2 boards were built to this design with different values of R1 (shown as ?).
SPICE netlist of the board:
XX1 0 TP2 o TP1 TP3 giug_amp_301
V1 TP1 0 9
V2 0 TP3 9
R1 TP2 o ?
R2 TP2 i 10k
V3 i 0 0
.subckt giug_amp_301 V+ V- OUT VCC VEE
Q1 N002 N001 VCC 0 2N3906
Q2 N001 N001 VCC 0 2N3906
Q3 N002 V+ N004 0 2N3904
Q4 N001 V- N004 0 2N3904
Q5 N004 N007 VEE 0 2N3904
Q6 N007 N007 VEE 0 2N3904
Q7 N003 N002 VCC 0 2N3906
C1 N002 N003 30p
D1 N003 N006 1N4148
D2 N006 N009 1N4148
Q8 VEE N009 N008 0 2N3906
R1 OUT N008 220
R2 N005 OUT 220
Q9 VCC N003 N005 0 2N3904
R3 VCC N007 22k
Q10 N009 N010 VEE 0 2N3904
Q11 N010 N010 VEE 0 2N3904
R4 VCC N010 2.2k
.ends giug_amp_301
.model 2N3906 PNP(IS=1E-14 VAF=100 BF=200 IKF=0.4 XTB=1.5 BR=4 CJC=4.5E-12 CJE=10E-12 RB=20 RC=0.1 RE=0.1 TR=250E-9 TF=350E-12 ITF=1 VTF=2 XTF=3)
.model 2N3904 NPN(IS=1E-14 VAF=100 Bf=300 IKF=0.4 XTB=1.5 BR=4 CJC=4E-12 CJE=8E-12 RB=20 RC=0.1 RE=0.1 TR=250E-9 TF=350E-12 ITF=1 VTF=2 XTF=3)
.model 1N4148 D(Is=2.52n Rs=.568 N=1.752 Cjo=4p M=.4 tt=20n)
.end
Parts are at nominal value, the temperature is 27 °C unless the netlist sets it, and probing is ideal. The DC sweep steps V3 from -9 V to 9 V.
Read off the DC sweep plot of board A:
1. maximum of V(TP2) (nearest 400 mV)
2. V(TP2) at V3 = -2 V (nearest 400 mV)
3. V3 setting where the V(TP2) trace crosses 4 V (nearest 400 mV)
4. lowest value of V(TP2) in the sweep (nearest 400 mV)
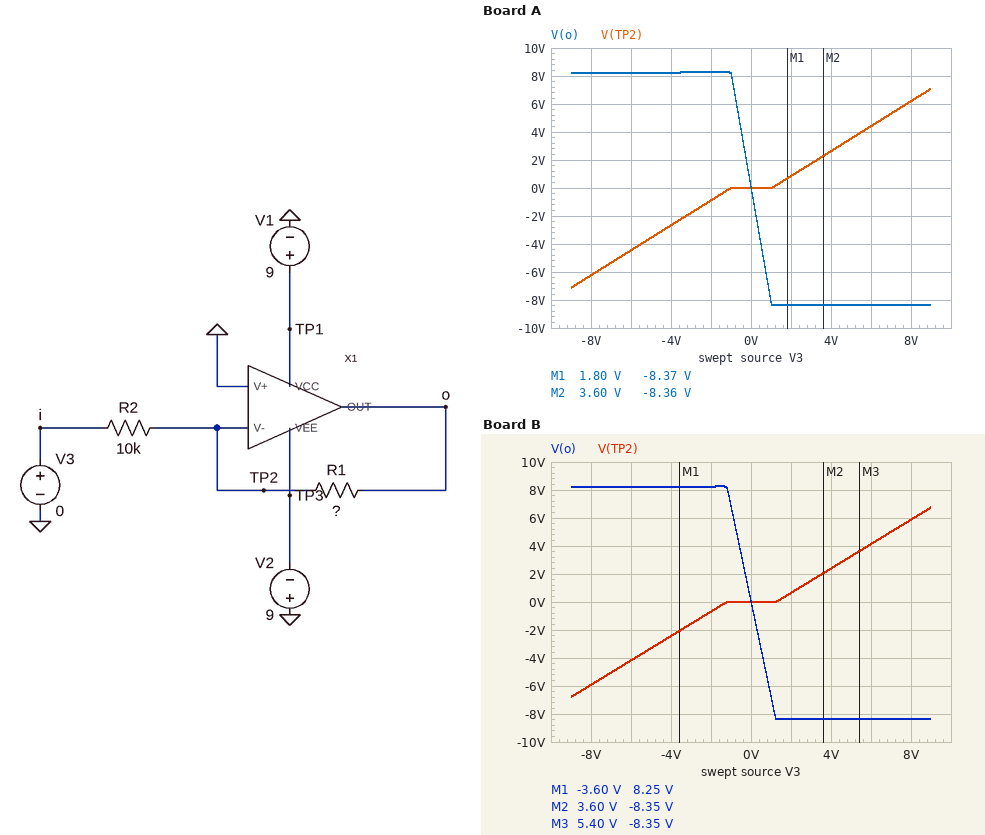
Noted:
7.2 V
-800 mV
5.6 V
-7.2 V
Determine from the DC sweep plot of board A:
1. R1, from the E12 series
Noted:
82 kΩ
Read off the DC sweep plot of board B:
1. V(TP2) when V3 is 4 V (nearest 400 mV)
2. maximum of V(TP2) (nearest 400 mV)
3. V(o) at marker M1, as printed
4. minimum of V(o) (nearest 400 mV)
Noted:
2.4 V
6.8 V
8.25 V
-8.4 V
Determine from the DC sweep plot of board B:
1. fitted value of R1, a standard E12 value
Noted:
68 kΩ
